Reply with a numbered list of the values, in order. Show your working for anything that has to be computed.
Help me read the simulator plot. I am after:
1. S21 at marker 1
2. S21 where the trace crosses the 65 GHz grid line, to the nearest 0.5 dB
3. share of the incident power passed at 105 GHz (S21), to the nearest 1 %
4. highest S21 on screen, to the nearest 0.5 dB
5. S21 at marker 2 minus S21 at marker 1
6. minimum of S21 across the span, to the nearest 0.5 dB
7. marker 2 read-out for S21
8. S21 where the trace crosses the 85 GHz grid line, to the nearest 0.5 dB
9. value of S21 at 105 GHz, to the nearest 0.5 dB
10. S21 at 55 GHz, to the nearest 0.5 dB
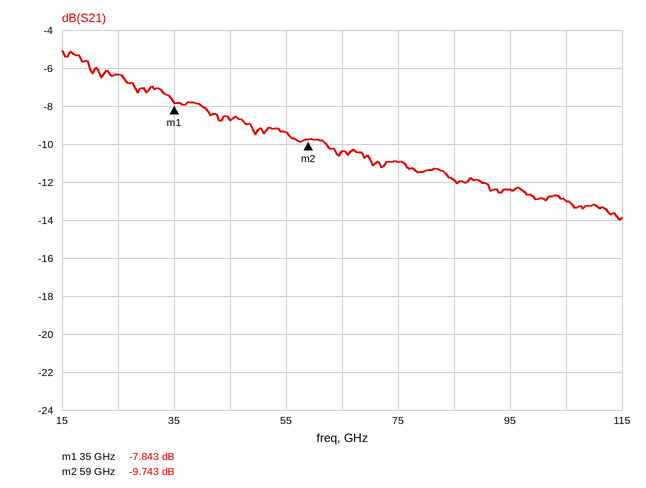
1. -7.843 dB
2. -10.5 dB
3. 10^(-13/10) ≈ 5 %
4. -5.0 dB
5. -9.743 − (-7.843) = -1.900 dB
6. -14.0 dB
7. -9.743 dB
8. -12.0 dB
9. -13.0 dB
10. -9.5 dB
